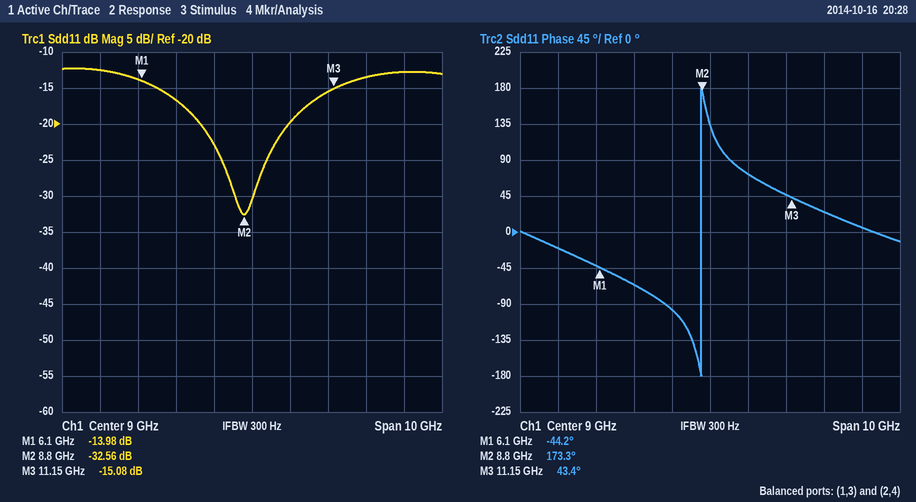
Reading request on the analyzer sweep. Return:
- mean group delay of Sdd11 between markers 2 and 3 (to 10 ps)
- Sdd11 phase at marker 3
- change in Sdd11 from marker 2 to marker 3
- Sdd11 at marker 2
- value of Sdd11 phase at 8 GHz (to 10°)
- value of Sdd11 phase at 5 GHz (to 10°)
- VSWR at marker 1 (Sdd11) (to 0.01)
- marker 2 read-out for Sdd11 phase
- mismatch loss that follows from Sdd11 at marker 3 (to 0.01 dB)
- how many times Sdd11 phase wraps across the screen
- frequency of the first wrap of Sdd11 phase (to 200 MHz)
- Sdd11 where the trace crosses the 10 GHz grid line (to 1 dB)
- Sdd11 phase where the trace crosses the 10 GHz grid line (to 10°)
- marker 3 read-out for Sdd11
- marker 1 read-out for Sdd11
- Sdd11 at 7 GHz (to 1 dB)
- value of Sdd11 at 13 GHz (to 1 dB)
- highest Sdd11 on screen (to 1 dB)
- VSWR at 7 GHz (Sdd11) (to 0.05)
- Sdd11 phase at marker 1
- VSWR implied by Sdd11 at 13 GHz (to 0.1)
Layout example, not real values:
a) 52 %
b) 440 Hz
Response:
a) 150 ps
b) 43.4°
c) 17.48 dB
d) -32.56 dB
e) -100°
f) -20°
g) 1.50
h) 173.3°
i) 0.14 dB
j) 1
k) 8.8 GHz
l) -20 dB
m) 70°
n) -15.08 dB
o) -13.98 dB
p) -17 dB
q) -13 dB
r) -12 dB
s) 1.35
t) -44.2°
u) 1.6
